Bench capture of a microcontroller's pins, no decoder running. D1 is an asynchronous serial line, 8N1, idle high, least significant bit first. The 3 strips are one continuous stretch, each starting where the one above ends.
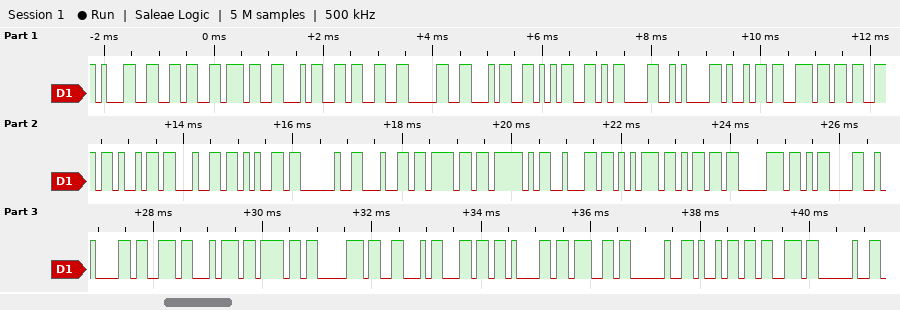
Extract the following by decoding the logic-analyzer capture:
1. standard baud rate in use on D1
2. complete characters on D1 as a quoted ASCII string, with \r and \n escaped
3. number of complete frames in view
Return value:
9600 baud
"16743045\r\ninside do_bump\r\nstopFlag is "
38
